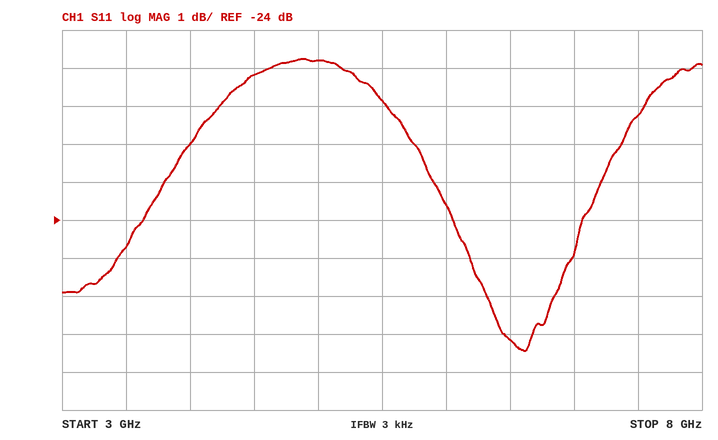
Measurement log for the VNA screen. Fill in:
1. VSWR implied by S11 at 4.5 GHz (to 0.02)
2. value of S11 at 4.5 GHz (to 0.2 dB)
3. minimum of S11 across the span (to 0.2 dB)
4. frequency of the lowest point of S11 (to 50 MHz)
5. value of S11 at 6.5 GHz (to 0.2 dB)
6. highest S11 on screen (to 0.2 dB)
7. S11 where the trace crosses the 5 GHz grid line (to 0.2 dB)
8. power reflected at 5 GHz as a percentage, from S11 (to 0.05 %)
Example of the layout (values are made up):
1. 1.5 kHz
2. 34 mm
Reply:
1. 1.22
2. -20.2 dB
3. -27.4 dB
4. 6.60 GHz
5. -27.2 dB
6. -19.8 dB
7. -19.8 dB
8. 1.05 %
